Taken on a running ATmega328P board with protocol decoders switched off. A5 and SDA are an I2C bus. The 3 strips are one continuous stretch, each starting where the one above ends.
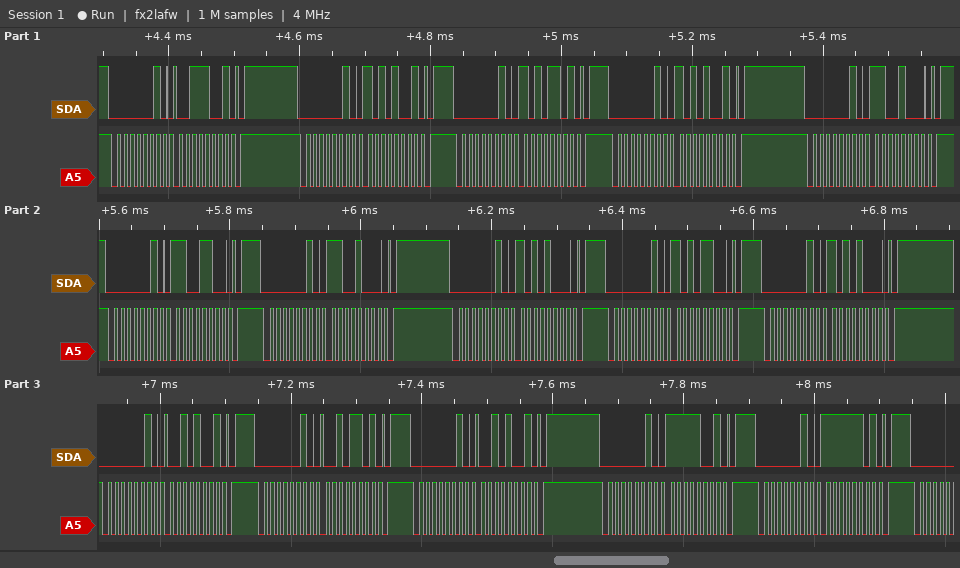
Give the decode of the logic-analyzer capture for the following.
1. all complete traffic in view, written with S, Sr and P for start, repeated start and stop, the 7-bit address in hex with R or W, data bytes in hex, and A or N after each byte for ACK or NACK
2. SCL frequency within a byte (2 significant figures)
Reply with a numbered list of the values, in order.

1. S 01W A 39 A P S 01W A A9 A P S 01W A AD A P S 01W A A9 A P S 01W A C8 A P S 01W A CC A P S 01W A C8 A P S 01W A A8 A P S 01W A AC A P S 01W A A8 A P S 01W A 29 A P S 01W A 2D A P S 01W A 29 A P S 01W A F9 A P S 01W A FD A P
2. 100 kHz
